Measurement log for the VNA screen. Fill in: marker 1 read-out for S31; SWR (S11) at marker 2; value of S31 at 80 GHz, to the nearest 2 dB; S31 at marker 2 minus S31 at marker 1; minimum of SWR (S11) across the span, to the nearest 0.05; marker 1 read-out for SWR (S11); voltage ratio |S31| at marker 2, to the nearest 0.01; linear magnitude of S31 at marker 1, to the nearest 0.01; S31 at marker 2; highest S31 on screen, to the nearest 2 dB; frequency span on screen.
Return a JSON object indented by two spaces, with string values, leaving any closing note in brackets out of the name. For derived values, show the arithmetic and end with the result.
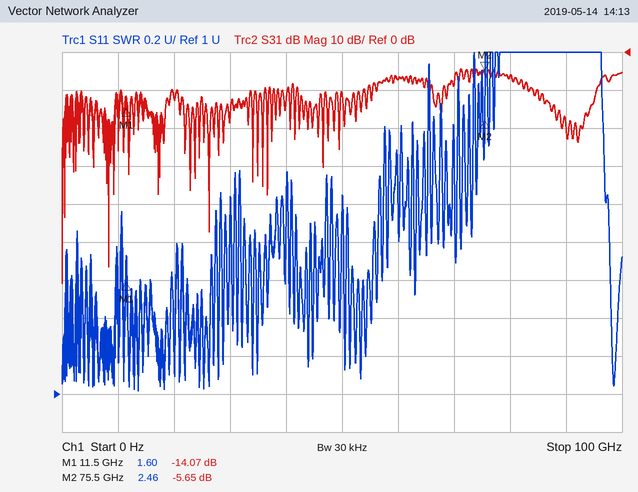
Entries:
{
  "marker 1 read-out for S31": "-14.07 dB",
  "SWR (S11) at marker 2": "2.46",
  "value of S31 at 80 GHz, to the nearest 2 dB": "-6 dB",
  "S31 at marker 2 minus S31 at marker 1": "-5.65 − (-14.07) = 8.42 dB",
  "minimum of SWR (S11) across the span, to the nearest 0.05": "1.00",
  "marker 1 read-out for SWR": "1.60",
  "voltage ratio |S31| at marker 2, to the nearest 0.01": "10^(-5.65/20) ≈ 0.52",
  "linear magnitude of S31 at marker 1, to the nearest 0.01": "10^(-14.07/20) ≈ 0.20",
  "S31 at marker 2": "-5.65 dB",
  "highest S31 on screen, to the nearest 2 dB": "-4 dB",
  "frequency span on screen": "100 GHz"
}
